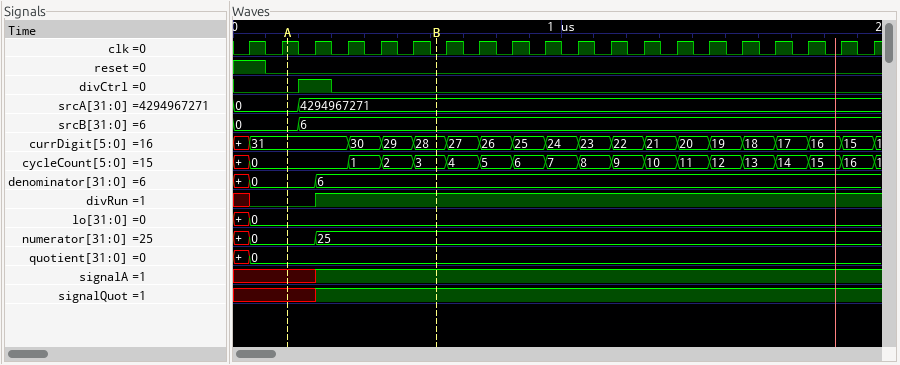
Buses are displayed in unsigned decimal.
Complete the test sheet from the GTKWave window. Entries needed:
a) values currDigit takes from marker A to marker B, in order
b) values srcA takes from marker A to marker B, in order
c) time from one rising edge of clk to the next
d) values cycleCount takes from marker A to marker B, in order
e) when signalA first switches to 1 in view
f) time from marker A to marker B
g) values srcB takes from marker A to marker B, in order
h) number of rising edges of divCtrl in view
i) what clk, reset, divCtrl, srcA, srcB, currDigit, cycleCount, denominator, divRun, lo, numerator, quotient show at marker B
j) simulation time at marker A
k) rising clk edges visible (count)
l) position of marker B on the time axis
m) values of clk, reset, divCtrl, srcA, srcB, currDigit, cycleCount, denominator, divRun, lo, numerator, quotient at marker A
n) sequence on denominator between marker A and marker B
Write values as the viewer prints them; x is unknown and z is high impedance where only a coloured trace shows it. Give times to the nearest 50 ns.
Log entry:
31, 30, 29, 28
0, 4294967271
100 ns
0, 1, 2, 3
250 ns
450 ns
0, 6
1
clk=0, reset=0, divCtrl=0, srcA=4294967271, srcB=6, currDigit=28, cycleCount=3, denominator=6, divRun=1, lo=0, numerator=25, quotient=0
150 ns
20
600 ns
clk=1, reset=0, divCtrl=0, srcA=0, srcB=0, currDigit=31, cycleCount=0, denominator=0, divRun=0, lo=0, numerator=0, quotient=0
0, 6
